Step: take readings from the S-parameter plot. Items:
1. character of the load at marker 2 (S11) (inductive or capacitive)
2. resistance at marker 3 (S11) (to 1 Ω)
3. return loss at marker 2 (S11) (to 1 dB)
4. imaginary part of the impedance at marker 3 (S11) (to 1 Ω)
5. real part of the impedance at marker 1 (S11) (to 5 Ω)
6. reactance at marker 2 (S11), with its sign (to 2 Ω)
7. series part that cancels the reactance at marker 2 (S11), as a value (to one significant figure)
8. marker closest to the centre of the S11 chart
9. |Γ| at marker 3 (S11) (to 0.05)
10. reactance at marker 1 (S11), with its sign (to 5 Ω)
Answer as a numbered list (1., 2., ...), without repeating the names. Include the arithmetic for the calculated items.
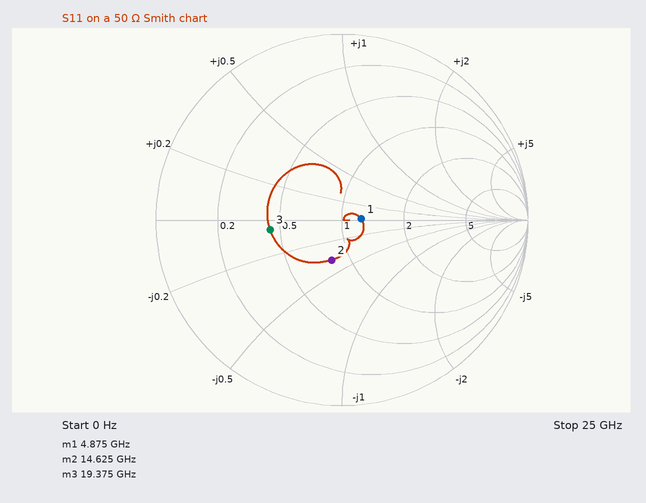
1. capacitive
2. 22 Ω
3. 13 dB
4. -3 Ω
5. 60 Ω
6. -18 Ω
7. L = 18 Ω/(2π × 14.625 GHz) ≈ 196 pH, so 200 pH to one significant figure
8. marker 1
9. 0.40
10. 0 Ω
